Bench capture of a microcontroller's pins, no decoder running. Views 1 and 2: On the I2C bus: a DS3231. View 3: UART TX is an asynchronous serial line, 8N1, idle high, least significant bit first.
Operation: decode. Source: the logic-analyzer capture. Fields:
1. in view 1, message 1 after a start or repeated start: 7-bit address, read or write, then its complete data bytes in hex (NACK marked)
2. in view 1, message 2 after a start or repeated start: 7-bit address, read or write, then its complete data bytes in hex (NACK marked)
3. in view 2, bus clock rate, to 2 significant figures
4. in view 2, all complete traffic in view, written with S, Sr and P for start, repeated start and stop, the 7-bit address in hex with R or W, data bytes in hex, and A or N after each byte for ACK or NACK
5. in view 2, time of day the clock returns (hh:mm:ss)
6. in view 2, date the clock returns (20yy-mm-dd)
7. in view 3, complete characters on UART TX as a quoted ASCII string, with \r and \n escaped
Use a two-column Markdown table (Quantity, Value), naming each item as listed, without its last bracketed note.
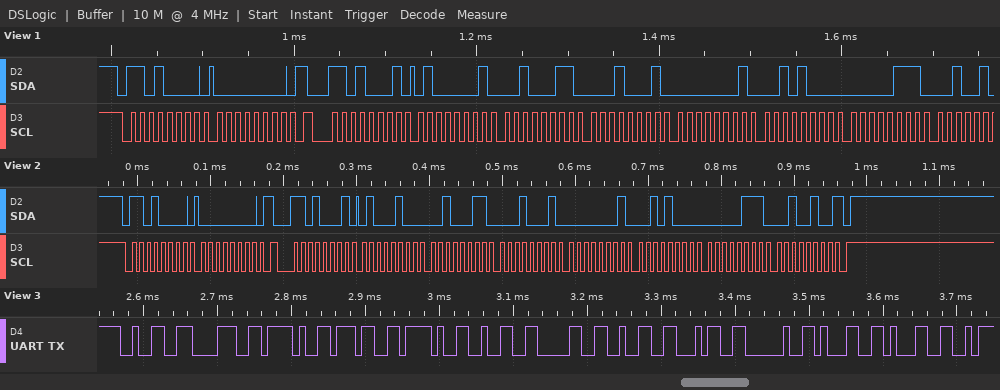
| Quantity | Value |
|---|---|
| in view 1, message 1 after a start or repeated start: 7-bit address, read or write, then its complete data bytes in hex | 0x68 write: 00 |
| in view 1, message 2 after a start or repeated start: 7-bit address, read or write, then its complete data bytes in hex | 0x68 read: 41 23 11 01 28 07 |
| in view 2, bus clock rate, to 2 significant figures | 100 kHz |
| in view 2, all complete traffic in view, written with S, Sr and P for start, repeated start and stop, the 7-bit address in hex with R or W, data bytes in hex, and A or N after each byte for ACK or NACK | S 68W A 00 A Sr 68R A 44 A 23 A 11 A 01 A 28 A 07 A 24 N P |
| in view 2, time of day the clock returns | 11:23:44 |
| in view 2, date the clock returns | 2024-07-28 |
| in view 3, complete characters on UART TX as a quoted ASCII string, with \r and \n escaped | "28/7/2024 11" |
